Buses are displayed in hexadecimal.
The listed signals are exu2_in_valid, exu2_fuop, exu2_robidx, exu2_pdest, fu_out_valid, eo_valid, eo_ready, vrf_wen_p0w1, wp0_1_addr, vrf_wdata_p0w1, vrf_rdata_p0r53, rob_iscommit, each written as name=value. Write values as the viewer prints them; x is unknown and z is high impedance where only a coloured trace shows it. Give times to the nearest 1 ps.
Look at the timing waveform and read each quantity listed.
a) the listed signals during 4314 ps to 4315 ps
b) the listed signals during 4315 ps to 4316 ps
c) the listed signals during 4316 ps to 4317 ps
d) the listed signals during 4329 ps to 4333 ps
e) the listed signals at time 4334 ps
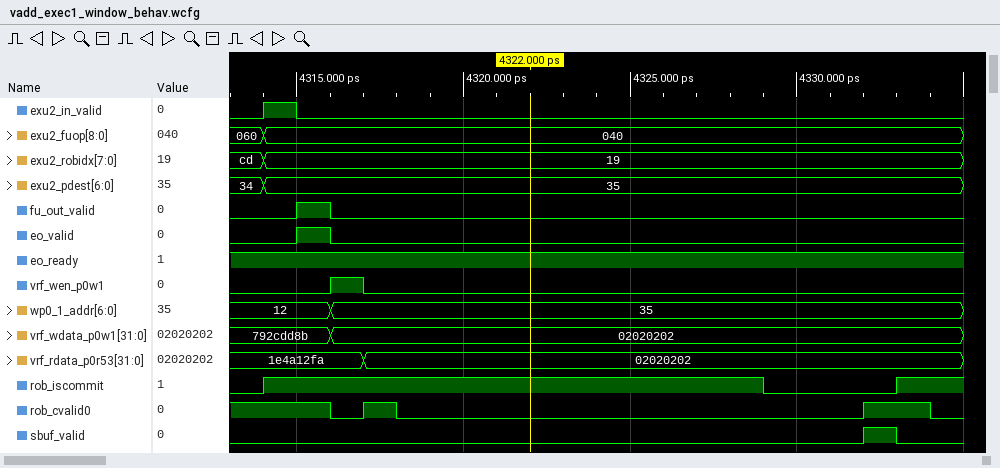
exu2_in_valid=1, exu2_fuop=040, exu2_robidx=19, exu2_pdest=35, fu_out_valid=0, eo_valid=0, eo_ready=1, vrf_wen_p0w1=0, wp0_1_addr=12, vrf_wdata_p0w1=792cdd8b, vrf_rdata_p0r53=1e4a12fa, rob_iscommit=1
exu2_in_valid=0, exu2_fuop=040, exu2_robidx=19, exu2_pdest=35, fu_out_valid=1, eo_valid=1, eo_ready=1, vrf_wen_p0w1=0, wp0_1_addr=12, vrf_wdata_p0w1=792cdd8b, vrf_rdata_p0r53=1e4a12fa, rob_iscommit=1
exu2_in_valid=0, exu2_fuop=040, exu2_robidx=19, exu2_pdest=35, fu_out_valid=0, eo_valid=0, eo_ready=1, vrf_wen_p0w1=1, wp0_1_addr=35, vrf_wdata_p0w1=02020202, vrf_rdata_p0r53=1e4a12fa, rob_iscommit=1
exu2_in_valid=0, exu2_fuop=040, exu2_robidx=19, exu2_pdest=35, fu_out_valid=0, eo_valid=0, eo_ready=1, vrf_wen_p0w1=0, wp0_1_addr=35, vrf_wdata_p0w1=02020202, vrf_rdata_p0r53=02020202, rob_iscommit=0
exu2_in_valid=0, exu2_fuop=040, exu2_robidx=19, exu2_pdest=35, fu_out_valid=0, eo_valid=0, eo_ready=1, vrf_wen_p0w1=0, wp0_1_addr=35, vrf_wdata_p0w1=02020202, vrf_rdata_p0r53=02020202, rob_iscommit=1
